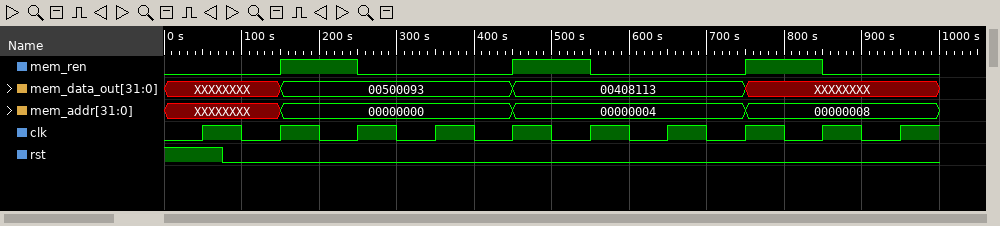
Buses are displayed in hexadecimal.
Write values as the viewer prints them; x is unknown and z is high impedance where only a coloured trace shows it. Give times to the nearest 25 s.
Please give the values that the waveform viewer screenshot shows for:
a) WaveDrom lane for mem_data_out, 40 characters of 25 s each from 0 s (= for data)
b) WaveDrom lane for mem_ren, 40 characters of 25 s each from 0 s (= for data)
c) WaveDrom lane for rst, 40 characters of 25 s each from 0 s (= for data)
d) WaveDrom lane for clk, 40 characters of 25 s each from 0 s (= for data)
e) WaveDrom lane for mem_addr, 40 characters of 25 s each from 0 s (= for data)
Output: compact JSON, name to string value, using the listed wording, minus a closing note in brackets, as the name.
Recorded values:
{"WaveDrom lane for mem_data_out, 40 characters of 25 s each from 0 s": "{name: 'mem_data_out', wave: 'x.....=...........=...........x.........', data: '00500093 00408113'}", "WaveDrom lane for mem_ren, 40 characters of 25 s each from 0 s": "{name: 'mem_ren', wave: '0.....1...0.......1...0.......1...0.....'}", "WaveDrom lane for rst, 40 characters of 25 s each from 0 s": "{name: 'rst', wave: '1..0....................................'}", "WaveDrom lane for clk, 40 characters of 25 s each from 0 s": "{name: 'clk', wave: '0.1.0.1.0.1.0.1.0.1.0.1.0.1.0.1.0.1.0.1.'}", "WaveDrom lane for mem_addr, 40 characters of 25 s each from 0 s": "{name: 'mem_addr', wave: 'x.....=...........=...........=.........', data: '00000000 00000004 00000008'}"}
